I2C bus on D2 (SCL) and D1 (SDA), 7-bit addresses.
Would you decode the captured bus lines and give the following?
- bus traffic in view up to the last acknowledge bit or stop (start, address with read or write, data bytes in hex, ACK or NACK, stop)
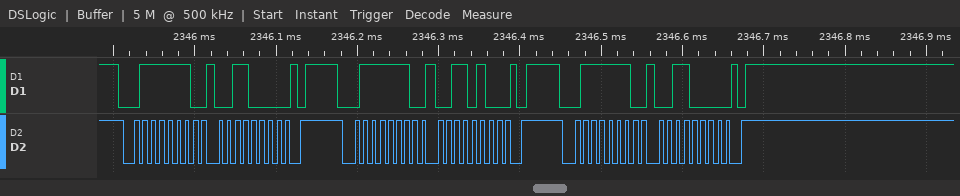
start, address 3F write ACK, 30 ACK, stop, start, address 3F write ACK, 34 ACK, stop, start, address 3F write ACK, 30 ACK, stop
